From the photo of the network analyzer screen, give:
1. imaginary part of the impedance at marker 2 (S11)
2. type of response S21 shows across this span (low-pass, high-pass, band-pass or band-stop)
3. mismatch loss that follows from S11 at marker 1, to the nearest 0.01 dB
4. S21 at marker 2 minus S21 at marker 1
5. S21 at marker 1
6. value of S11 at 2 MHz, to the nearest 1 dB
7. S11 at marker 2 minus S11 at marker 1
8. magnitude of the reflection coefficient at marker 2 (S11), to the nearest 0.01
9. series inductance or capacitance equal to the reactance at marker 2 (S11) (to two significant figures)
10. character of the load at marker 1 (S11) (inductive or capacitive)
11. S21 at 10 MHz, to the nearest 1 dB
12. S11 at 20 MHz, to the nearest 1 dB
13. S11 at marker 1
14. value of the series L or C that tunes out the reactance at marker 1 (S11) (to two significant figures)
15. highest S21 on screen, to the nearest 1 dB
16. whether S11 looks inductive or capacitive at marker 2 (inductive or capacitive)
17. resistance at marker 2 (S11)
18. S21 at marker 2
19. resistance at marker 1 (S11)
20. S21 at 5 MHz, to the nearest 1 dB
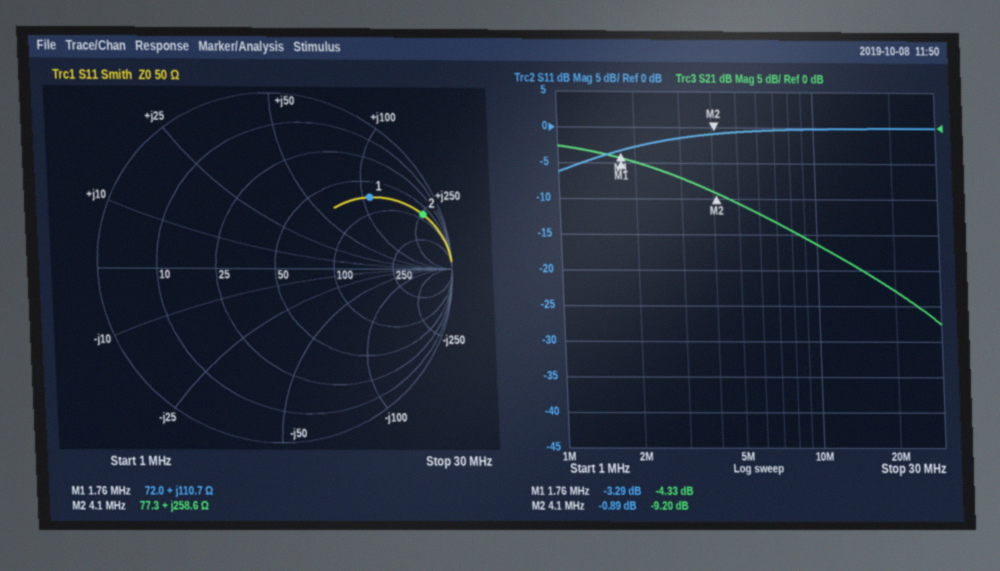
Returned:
+258.6 Ω
low-pass
2.75 dB
-4.87 dB
-4.33 dB
-3 dB
2.40 dB
0.90
10 µH
inductive
-16 dB
0 dB
-3.29 dB
820 pF
-3 dB
inductive
77.3 Ω
-9.20 dB
72.0 Ω
-11 dB
